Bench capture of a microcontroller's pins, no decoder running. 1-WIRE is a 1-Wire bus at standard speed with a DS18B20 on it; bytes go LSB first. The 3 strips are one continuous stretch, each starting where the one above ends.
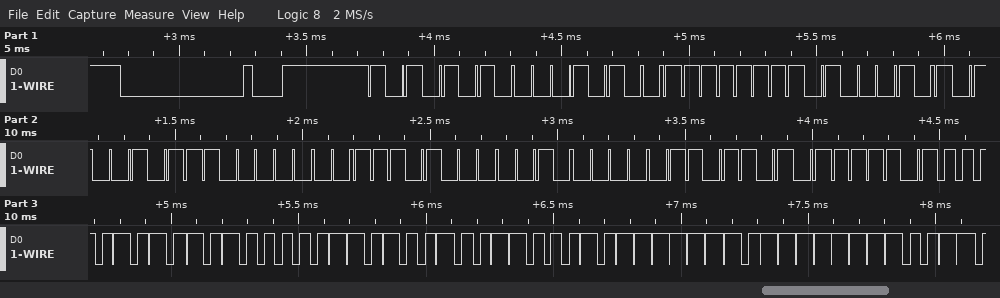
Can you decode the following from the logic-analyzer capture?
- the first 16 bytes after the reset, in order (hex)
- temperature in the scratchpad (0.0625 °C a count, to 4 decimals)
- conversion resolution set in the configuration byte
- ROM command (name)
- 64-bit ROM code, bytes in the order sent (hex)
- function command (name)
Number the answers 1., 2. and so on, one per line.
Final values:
1. 55 28 FF A2 D2 01 17 04 B6 BE 50 05 4B 46 7F FF
2. 85.0000 °C
3. 12 bits
4. Match ROM
5. 28 FF A2 D2 01 17 04 B6
6. Read Scratchpad
